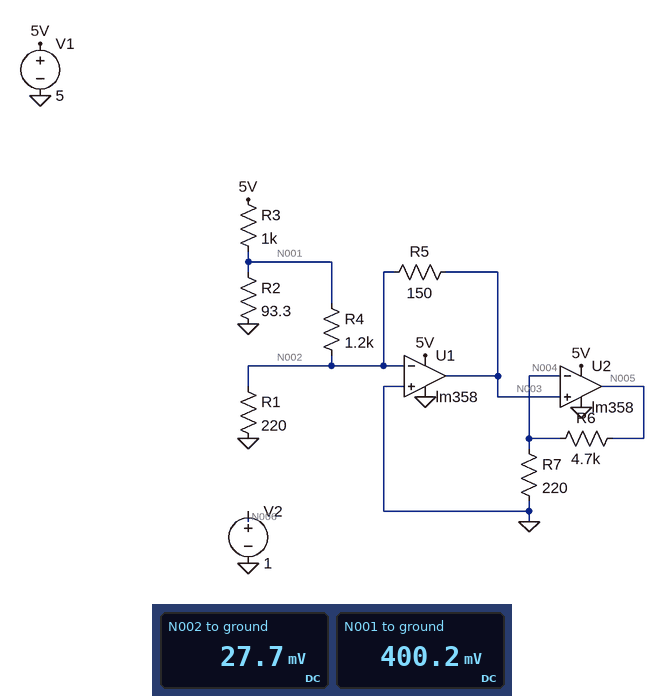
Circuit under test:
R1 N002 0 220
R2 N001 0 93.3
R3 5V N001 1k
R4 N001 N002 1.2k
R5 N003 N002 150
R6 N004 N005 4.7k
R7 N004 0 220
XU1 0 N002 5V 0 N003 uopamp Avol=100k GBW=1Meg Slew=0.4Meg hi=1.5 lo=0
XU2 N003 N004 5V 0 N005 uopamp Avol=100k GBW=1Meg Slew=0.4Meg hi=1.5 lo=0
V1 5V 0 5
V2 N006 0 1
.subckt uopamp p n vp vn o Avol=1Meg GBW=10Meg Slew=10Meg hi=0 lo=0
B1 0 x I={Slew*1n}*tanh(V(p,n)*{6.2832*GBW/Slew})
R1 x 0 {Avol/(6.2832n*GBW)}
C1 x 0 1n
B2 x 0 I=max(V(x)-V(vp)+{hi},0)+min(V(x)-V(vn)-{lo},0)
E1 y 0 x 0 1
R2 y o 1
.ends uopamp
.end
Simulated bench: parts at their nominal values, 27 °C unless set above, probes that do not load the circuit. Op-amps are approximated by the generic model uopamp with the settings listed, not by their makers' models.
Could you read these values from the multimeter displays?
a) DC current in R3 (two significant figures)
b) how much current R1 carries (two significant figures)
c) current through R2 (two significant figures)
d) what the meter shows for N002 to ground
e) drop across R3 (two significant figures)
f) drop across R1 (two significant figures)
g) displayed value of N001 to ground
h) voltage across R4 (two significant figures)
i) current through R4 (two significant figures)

4.6 mA
130 µA
4.3 mA
27.7 mV
4.6 V
28 mV
400.2 mV
370 mV
310 µA
